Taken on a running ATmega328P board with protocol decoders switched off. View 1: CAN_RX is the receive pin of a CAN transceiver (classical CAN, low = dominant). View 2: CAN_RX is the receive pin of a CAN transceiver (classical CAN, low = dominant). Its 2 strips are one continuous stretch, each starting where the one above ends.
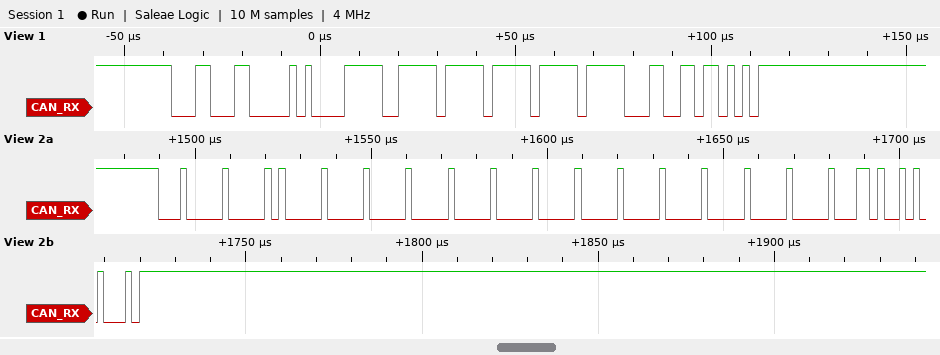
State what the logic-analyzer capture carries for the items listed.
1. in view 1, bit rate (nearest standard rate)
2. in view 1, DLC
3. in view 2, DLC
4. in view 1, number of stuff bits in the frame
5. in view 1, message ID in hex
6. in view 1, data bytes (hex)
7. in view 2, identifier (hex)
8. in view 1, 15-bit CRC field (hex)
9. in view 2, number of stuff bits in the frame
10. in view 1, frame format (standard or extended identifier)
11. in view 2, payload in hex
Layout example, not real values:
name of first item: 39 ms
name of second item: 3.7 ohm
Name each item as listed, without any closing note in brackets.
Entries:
in view 1, bit rate: 500 kbit/s
in view 1, DLC: 4
in view 2, DLC: 8
in view 1, number of stuff bits in the frame: 7
in view 1, message ID in hex: 0x18C
in view 1, data bytes: 3E FF FF FF
in view 2, identifier: 0x100
in view 1, 15-bit CRC field: 0x4CDA
in view 2, number of stuff bits in the frame: 15
in view 1, frame format: standard
in view 2, payload in hex: 00 00 00 00 00 00 00 00
